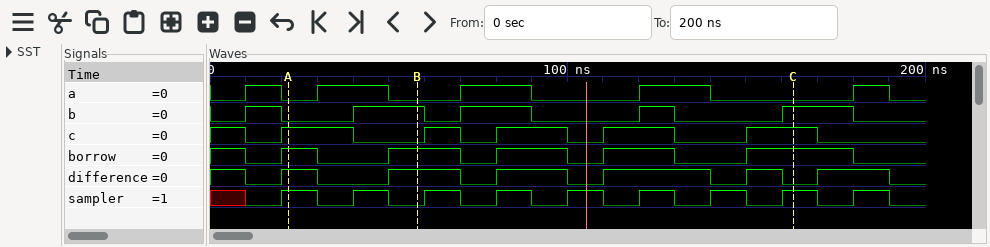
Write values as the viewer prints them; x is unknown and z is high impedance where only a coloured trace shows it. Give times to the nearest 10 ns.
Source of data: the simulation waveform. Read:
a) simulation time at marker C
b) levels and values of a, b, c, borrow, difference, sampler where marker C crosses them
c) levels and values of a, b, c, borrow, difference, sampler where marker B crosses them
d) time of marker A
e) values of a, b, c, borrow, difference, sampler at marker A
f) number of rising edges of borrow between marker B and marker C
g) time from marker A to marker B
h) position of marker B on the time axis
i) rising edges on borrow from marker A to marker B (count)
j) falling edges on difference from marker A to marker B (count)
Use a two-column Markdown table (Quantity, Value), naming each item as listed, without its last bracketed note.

| Quantity | Value |
|---|---|
| simulation time at marker C | 160 ns |
| levels and values of a, b, c, borrow, difference, sampler where marker C crosses them | a=0, b=1, c=1, borrow=1, difference=0, sampler=1 |
| levels and values of a, b, c, borrow, difference, sampler where marker B crosses them | a=0, b=1, c=0, borrow=1, difference=1, sampler=0 |
| time of marker A | 20 ns |
| values of a, b, c, borrow, difference, sampler at marker A | a=0, b=0, c=1, borrow=1, difference=1, sampler=1 |
| number of rising edges of borrow between marker B and marker C | 3 |
| time from marker A to marker B | 40 ns |
| position of marker B on the time axis | 60 ns |
| rising edges on borrow from marker A to marker B | 1 |
| falling edges on difference from marker A to marker B | 1 |
